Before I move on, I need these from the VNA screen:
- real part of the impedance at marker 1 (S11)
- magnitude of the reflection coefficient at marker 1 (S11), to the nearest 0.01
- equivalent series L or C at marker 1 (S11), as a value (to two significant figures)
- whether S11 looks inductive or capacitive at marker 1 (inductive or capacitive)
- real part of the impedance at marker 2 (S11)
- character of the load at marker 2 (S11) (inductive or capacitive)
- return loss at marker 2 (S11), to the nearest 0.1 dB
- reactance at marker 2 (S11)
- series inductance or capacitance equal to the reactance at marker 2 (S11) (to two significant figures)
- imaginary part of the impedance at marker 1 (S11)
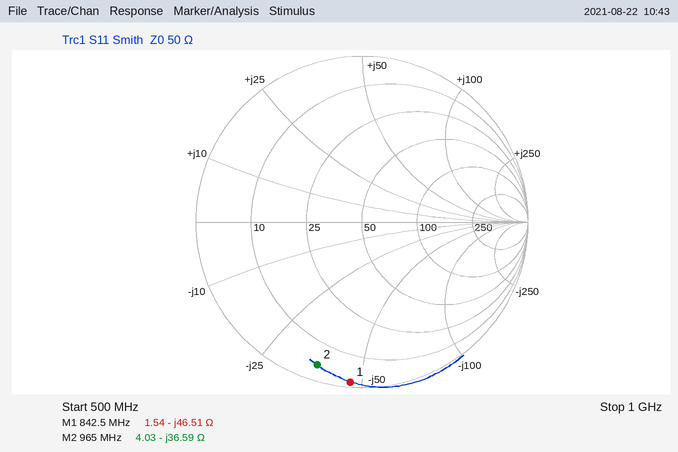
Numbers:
1.54 Ω
0.97
4.1 pF
capacitive
4.03 Ω
capacitive
0.9 dB
-36.59 Ω
4.5 pF
-46.51 Ω
